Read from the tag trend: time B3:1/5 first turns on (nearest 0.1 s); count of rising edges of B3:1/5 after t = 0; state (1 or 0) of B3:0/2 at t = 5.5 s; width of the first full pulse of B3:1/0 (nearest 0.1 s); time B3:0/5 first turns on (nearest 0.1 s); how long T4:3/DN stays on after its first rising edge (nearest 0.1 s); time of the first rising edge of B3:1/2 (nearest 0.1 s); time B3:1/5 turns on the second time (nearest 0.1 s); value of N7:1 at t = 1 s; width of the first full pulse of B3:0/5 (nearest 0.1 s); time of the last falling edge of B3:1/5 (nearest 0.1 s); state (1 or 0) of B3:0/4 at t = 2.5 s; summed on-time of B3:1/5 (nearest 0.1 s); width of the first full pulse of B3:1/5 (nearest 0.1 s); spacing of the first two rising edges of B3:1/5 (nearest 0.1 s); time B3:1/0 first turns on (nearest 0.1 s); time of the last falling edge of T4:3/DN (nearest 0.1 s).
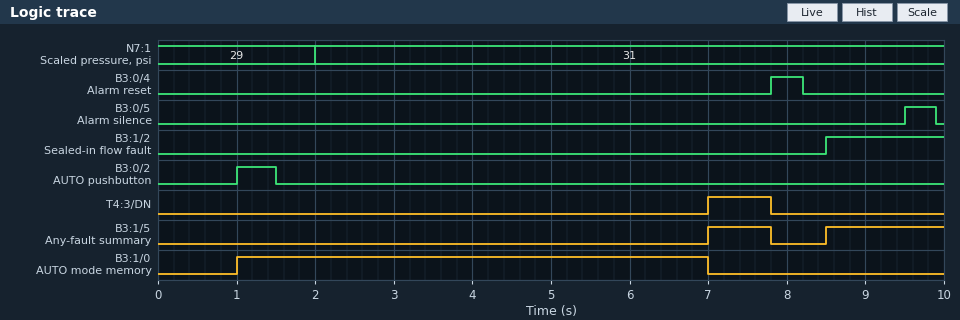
7.0 s
2
0
6.0 s
9.5 s
0.8 s
8.5 s
8.5 s
29
0.4 s
7.8 s
0
2.3 s
0.8 s
1.5 s
1.0 s
7.8 s
